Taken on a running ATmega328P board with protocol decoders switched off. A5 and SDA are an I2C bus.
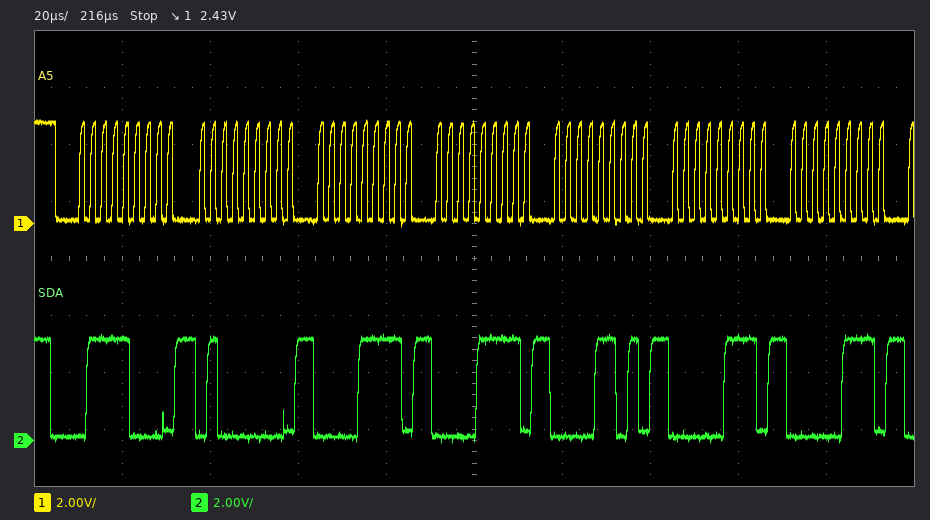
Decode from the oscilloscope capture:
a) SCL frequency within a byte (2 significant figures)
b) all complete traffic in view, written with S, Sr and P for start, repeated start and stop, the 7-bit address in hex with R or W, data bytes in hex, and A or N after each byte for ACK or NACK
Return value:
400 kHz
S 3CW A 40 A 0F A 0F A 0D A 07 A 07 A
